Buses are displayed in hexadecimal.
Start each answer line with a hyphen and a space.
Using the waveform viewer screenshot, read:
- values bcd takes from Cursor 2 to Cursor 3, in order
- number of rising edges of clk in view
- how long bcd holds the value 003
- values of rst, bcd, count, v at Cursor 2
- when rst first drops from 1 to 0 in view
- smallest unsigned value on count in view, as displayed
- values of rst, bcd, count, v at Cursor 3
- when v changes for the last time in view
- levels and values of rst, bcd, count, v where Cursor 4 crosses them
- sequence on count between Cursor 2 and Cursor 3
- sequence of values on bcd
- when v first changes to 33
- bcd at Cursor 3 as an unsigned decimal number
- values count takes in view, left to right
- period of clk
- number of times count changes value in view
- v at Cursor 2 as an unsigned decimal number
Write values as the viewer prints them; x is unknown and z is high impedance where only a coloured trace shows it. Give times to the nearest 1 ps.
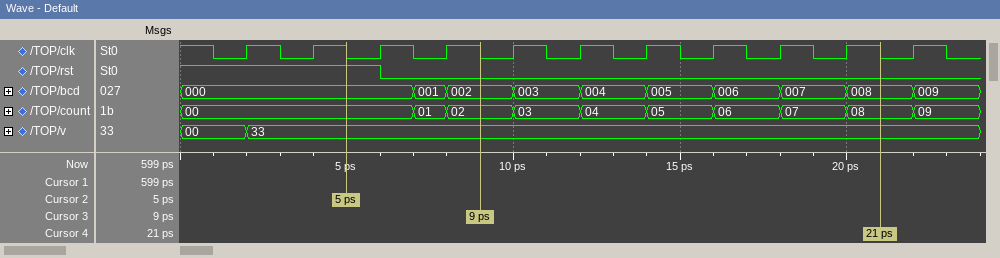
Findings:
- 000, 001, 002
- 11
- 2 ps
- rst=1, bcd=000, count=00, v=33
- 6 ps
- 00
- rst=0, bcd=002, count=02, v=33
- 2 ps
- rst=0, bcd=008, count=08, v=33
- 00, 01, 02
- 000, 001, 002, 003, 004, 005, 006, 007, 008, 009
- 2 ps
- 2
- 00, 01, 02, 03, 04, 05, 06, 07, 08, 09
- 2 ps
- 9
- 51
